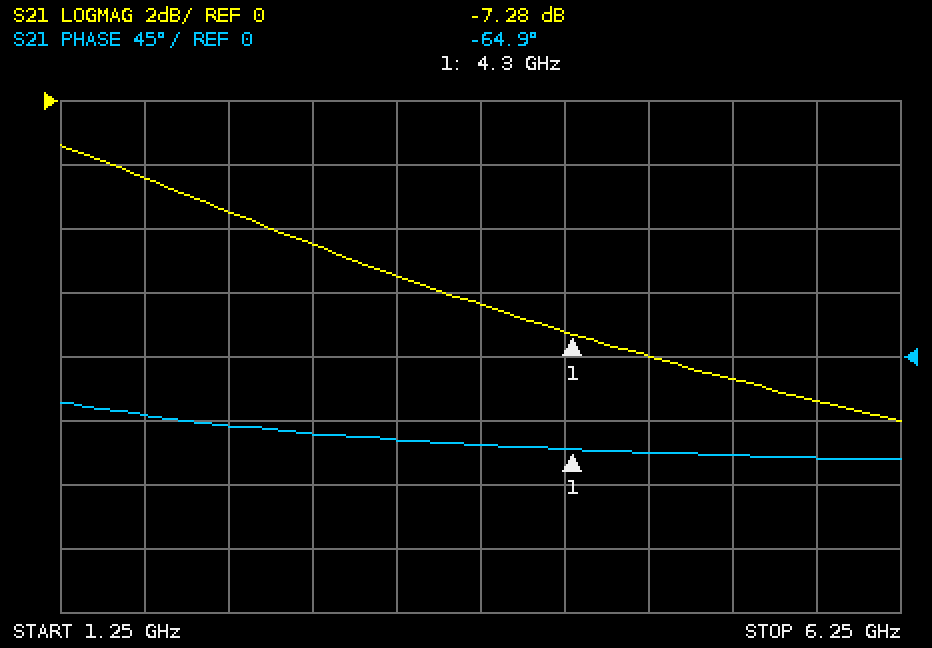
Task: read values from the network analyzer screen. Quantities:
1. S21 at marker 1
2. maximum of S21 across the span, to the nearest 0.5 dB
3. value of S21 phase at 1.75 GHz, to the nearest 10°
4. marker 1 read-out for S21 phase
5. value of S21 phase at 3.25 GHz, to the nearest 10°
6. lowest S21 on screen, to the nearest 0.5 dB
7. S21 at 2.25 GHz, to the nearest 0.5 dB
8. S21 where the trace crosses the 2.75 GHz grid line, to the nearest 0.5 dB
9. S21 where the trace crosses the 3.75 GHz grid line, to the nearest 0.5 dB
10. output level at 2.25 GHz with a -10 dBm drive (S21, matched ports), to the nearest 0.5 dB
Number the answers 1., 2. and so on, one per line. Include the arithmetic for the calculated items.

1. -7.28 dB
2. -1.5 dB
3. -40°
4. -64.9°
5. -60°
6. -10.0 dB
7. -3.5 dB
8. -4.5 dB
9. -6.5 dB
10. -10 dBm + (-3.5 dB) = -13.5 dBm
